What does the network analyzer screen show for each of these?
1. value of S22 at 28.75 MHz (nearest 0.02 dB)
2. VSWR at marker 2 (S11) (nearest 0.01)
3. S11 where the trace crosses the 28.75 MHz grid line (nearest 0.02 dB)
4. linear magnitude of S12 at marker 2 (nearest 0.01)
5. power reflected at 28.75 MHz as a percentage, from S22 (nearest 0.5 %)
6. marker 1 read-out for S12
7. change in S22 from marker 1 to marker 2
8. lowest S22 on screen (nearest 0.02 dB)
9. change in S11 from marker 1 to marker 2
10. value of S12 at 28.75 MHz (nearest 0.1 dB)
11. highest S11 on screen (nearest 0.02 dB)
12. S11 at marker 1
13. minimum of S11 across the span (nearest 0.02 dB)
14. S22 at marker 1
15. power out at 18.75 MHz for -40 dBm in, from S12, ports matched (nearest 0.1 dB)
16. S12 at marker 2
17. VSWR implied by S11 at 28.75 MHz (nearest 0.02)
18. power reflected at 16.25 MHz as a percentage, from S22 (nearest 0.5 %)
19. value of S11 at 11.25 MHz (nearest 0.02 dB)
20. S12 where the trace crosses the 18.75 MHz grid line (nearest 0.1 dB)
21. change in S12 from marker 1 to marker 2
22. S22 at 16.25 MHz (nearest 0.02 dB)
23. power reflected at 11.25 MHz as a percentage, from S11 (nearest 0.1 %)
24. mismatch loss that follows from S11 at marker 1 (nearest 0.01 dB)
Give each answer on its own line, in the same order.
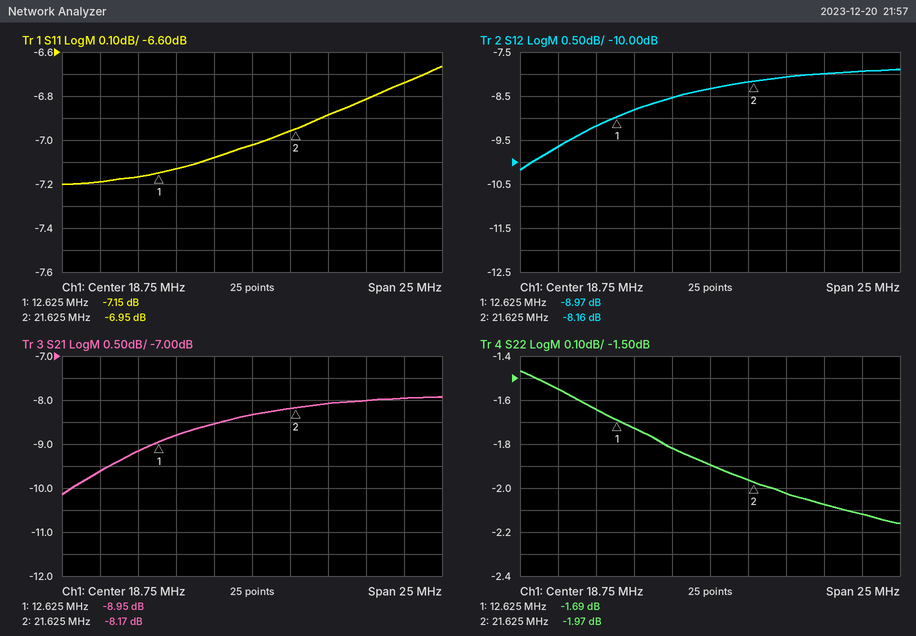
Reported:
-2.12 dB
2.63
-6.74 dB
0.39
61.5 %
-8.97 dB
-0.28 dB
-2.16 dB
0.20 dB
-7.9 dB
-6.66 dB
-7.15 dB
-7.20 dB
-1.69 dB
-48.3 dBm
-8.16 dB
2.70
66.0 %
-7.16 dB
-8.3 dB
0.81 dB
-1.82 dB
19.2 %
0.93 dB
